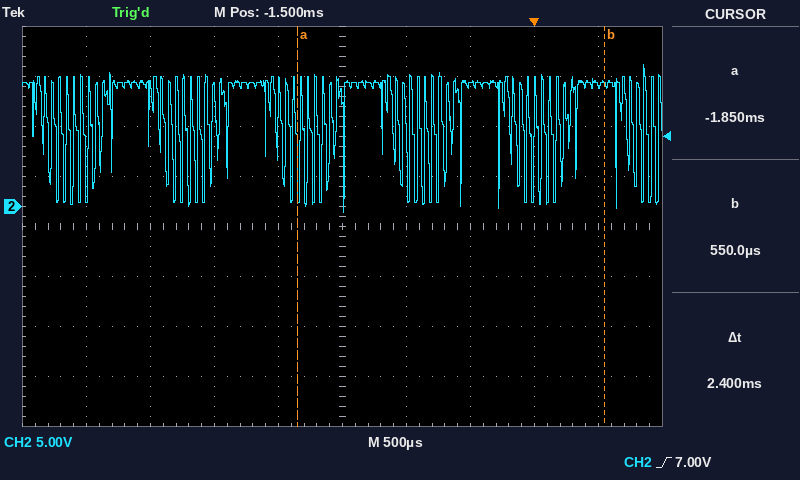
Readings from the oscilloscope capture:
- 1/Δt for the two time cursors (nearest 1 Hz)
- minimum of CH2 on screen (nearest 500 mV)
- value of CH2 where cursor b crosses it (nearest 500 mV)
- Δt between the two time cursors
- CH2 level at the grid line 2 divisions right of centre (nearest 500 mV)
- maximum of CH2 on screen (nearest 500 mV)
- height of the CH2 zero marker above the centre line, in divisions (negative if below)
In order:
417 Hz
-500 mV
12.0 V
2.4 ms
12.0 V
14.0 V
+0.4 div
